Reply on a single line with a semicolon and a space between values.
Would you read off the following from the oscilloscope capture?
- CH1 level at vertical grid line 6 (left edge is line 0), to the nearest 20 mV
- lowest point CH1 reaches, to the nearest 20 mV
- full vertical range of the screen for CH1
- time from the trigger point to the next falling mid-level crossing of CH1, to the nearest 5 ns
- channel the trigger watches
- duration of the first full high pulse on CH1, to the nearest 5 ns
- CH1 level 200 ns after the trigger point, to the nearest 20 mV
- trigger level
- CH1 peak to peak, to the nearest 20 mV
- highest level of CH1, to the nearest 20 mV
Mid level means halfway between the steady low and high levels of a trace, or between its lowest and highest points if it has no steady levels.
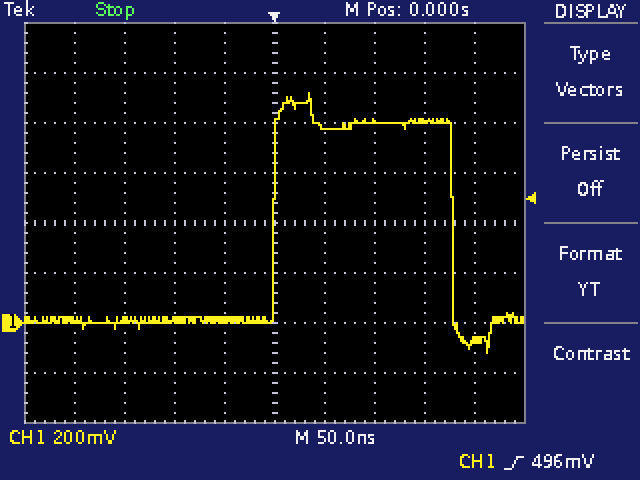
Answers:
780 mV; -120 mV; 1.6 V; 180 ns; CH1; 180 ns; -80 mV; 496 mV; 1.04 V; 920 mV
